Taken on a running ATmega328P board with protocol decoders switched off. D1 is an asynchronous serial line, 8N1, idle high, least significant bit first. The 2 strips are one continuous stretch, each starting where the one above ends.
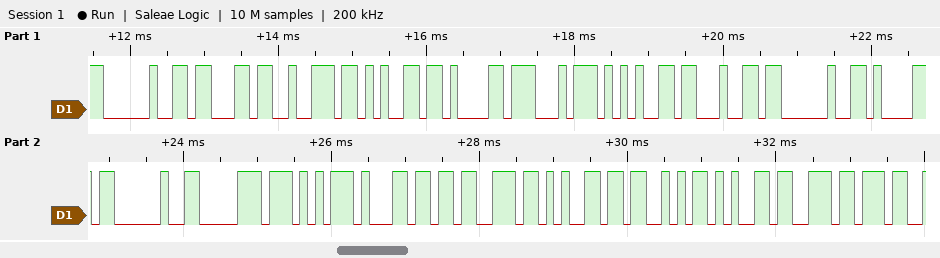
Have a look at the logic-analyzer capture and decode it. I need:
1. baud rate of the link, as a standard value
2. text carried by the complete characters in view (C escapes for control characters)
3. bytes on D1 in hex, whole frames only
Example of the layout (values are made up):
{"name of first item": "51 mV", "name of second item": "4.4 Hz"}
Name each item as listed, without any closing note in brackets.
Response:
{"baud rate of the link, as a standard value": "9600 baud", "text carried by the complete characters in view": "\" created a pulseSen\"", "bytes on D1 in hex, whole frames only": "20 63 72 65 61 74 65 64 20 61 20 70 75 6C 73 65 53 65 6E"}
